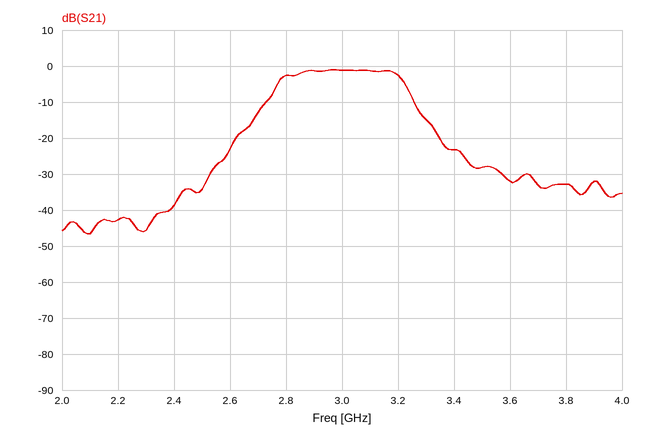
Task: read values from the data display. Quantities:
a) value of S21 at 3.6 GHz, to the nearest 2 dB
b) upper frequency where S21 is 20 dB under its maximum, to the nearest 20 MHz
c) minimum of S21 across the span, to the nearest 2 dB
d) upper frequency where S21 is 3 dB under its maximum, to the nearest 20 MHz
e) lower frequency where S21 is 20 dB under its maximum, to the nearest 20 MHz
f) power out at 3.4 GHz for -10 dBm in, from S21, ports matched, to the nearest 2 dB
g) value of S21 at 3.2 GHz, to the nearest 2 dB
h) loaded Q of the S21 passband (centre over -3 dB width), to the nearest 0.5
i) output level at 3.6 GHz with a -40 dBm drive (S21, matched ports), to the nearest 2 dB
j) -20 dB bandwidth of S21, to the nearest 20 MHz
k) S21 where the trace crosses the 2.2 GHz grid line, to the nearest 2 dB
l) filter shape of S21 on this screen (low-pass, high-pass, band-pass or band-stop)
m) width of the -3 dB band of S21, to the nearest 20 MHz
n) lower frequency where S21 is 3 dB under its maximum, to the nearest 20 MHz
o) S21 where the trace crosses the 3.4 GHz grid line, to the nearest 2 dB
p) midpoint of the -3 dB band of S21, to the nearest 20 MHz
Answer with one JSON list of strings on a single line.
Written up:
["-32 dB", "3.36 GHz", "-46 dB", "3.22 GHz", "2.62 GHz", "-34 dBm", "-2 dB", "7.0", "-72 dBm", "740 MHz", "-42 dB", "band-pass", "440 MHz", "2.78 GHz", "-24 dB", "3.00 GHz"]
